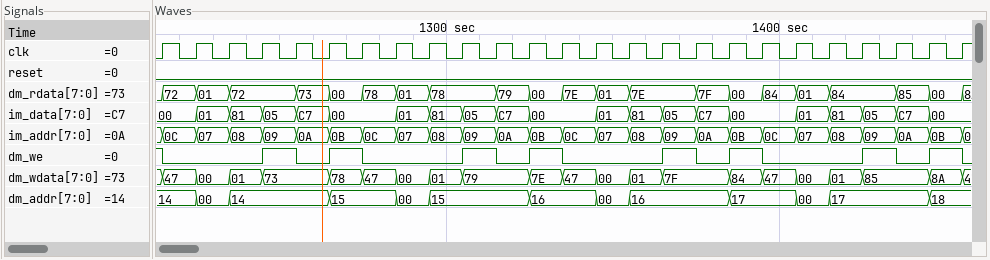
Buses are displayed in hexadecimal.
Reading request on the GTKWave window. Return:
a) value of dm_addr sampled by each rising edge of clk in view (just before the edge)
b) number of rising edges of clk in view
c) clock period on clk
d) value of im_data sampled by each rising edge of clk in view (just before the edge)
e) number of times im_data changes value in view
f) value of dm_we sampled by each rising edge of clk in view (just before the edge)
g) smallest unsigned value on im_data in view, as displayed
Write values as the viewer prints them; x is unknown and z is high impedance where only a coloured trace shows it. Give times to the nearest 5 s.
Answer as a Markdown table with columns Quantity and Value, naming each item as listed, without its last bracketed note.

| Quantity | Value |
|---|---|
| value of dm_addr sampled by each rising edge of clk in view | 14, 14, 00, 14, 14, 14, 15, 15, 00, 15, 15, 15, 16, 16, 00, 16, 16, 16, 17, 17, 00, 17, 17, 17, 18 |
| number of rising edges of clk in view | 25 |
| clock period on clk | 10 s |
| value of im_data sampled by each rising edge of clk in view | 00, 00, 01, 81, 05, C7, 00, 00, 01, 81, 05, C7, 00, 00, 01, 81, 05, C7, 00, 00, 01, 81, 05, C7, 00 |
| number of times im_data changes value in view | 20 |
| value of dm_we sampled by each rising edge of clk in view | 1 0 0 0 1 0 1 0 0 0 1 0 1 0 0 0 1 0 1 0 0 0 1 0 1 |
| smallest unsigned value on im_data in view, as displayed | 00 |
